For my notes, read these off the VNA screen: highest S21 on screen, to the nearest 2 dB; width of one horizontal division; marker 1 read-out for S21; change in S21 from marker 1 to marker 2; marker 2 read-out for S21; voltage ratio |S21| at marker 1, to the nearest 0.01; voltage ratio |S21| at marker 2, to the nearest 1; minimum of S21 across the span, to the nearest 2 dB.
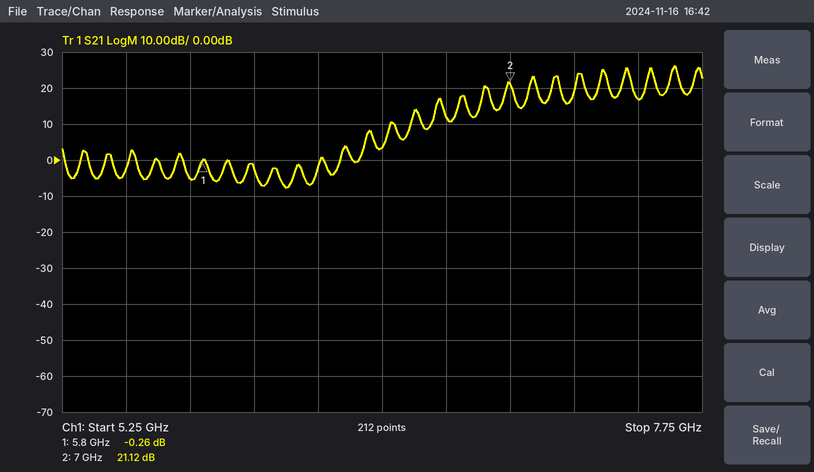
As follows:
26 dB
250 MHz
-0.26 dB
21.38 dB
21.12 dB
0.97
11
-8 dB
